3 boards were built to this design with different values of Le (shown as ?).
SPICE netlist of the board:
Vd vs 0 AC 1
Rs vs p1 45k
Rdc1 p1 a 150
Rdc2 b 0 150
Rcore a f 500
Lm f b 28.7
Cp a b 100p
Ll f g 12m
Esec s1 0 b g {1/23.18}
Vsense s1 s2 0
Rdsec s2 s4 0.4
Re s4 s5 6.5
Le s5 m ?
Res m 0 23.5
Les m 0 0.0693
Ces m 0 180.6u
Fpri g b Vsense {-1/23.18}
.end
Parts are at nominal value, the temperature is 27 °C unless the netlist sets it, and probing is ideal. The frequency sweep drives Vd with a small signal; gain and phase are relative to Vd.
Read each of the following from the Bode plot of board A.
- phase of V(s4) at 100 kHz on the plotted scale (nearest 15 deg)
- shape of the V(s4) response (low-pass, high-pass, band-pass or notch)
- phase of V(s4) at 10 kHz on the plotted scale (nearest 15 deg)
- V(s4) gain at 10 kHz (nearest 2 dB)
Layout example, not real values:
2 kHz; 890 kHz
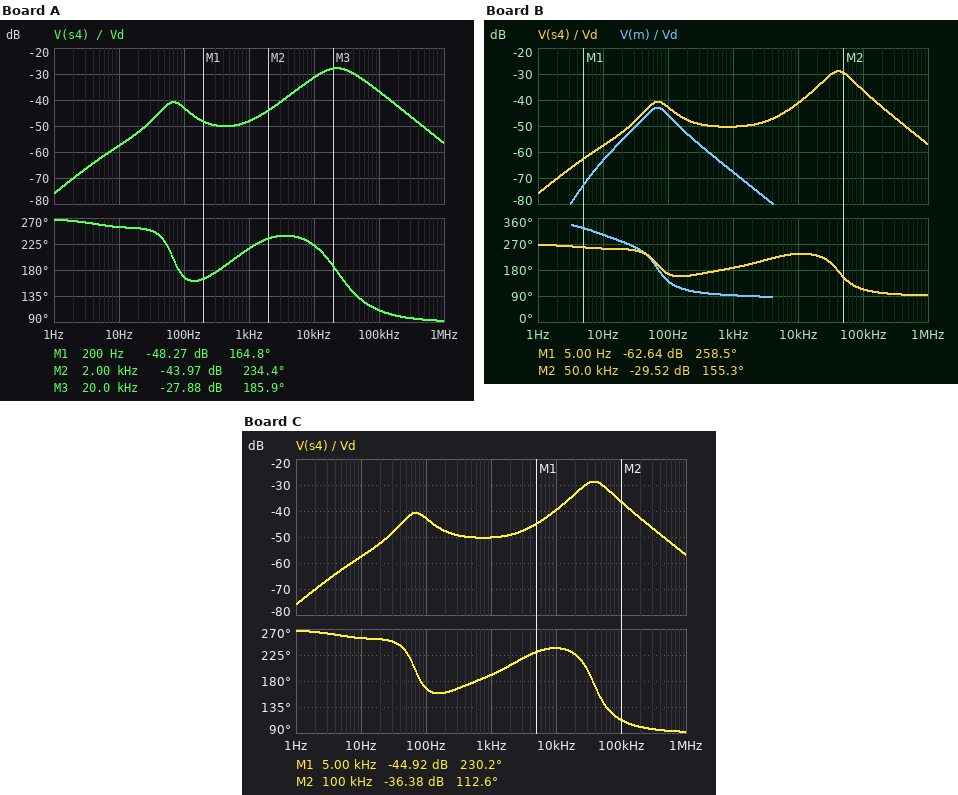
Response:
105 deg; band-pass; 225 deg; -32 dB
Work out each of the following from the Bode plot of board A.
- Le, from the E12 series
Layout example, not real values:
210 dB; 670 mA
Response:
1 mH
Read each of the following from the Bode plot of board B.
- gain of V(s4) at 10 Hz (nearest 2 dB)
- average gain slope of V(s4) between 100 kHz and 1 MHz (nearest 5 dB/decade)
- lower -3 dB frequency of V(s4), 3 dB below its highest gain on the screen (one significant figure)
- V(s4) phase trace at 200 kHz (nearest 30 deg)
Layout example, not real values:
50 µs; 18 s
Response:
-58 dB; -20 dB/decade; 30 kHz; 90 deg
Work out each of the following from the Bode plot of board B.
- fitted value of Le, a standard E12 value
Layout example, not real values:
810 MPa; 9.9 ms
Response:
270 µH
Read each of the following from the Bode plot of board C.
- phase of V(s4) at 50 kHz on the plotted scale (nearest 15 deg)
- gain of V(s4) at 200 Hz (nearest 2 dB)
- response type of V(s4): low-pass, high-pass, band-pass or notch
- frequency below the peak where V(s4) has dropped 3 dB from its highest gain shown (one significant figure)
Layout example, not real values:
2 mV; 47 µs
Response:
150 deg; -48 dB; band-pass; 20 kHz
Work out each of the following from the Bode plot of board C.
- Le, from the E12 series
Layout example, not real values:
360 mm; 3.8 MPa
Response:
330 µH
